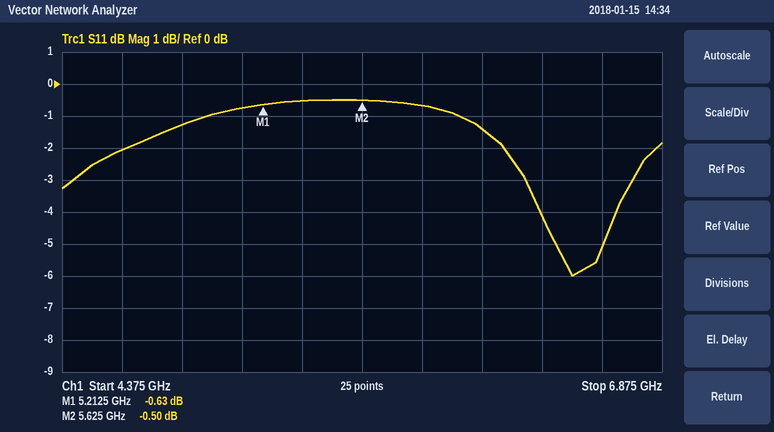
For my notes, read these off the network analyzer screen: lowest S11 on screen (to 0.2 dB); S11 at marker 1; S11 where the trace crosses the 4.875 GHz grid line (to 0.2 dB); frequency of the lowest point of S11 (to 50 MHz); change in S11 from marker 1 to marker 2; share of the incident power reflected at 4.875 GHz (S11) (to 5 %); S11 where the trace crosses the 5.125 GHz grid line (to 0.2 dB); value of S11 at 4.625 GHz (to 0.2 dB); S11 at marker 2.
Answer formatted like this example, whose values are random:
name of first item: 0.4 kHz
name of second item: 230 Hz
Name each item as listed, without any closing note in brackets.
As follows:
lowest S11 on screen: -6.0 dB
S11 at marker 1: -0.63 dB
S11 where the trace crosses the 4.875 GHz grid line: -1.2 dB
frequency of the lowest point of S11: 6.50 GHz
change in S11 from marker 1 to marker 2: 0.13 dB
share of the incident power reflected at 4.875 GHz (S11): 75 %
S11 where the trace crosses the 5.125 GHz grid line: -0.8 dB
value of S11 at 4.625 GHz: -2.0 dB
S11 at marker 2: -0.50 dB
